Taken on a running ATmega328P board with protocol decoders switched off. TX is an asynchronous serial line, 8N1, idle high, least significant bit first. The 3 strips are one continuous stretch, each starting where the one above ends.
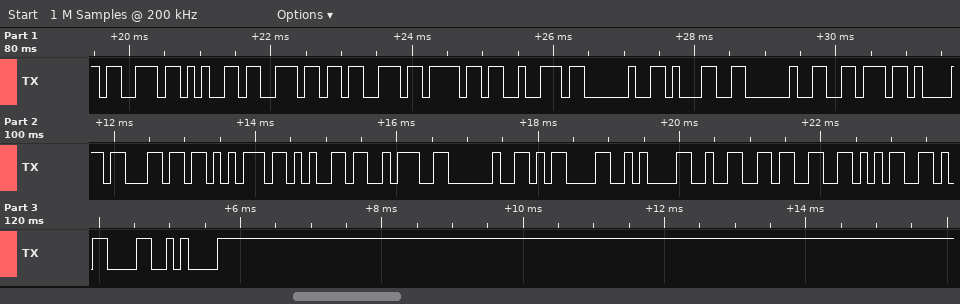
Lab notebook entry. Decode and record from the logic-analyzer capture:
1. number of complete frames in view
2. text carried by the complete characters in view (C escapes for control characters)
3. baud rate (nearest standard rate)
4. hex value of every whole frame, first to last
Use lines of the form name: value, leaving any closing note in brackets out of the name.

number of complete frames in view: 23
text carried by the complete characters in view: "sensor 1 value: \r\n235\r\n"
baud rate: 9600 baud
hex value of every whole frame, first to last: 73 65 6E 73 6F 72 20 31 20 76 61 6C 75 65 3A 20 0D 0A 32 33 35 0D 0A
